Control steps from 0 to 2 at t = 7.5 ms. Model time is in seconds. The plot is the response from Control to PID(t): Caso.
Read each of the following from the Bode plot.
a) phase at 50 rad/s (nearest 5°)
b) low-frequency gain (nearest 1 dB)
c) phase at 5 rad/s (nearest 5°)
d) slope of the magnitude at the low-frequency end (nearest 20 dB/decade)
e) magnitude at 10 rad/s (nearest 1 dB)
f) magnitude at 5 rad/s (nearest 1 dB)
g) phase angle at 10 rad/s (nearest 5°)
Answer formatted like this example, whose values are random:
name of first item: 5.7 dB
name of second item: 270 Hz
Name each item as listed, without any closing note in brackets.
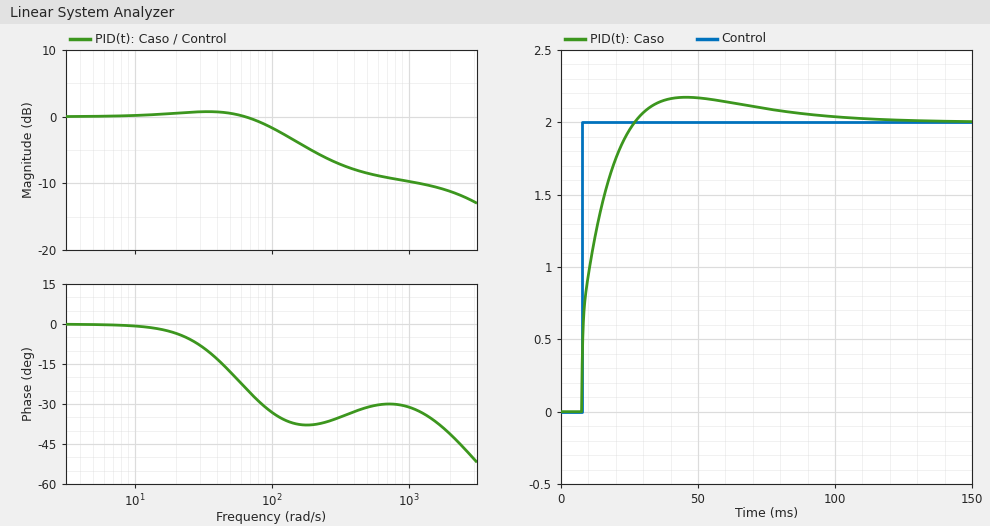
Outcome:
phase at 50 rad/s: -20°
low-frequency gain: 0 dB
phase at 5 rad/s: 0°
slope of the magnitude at the low-frequency end: 0 dB/decade
magnitude at 10 rad/s: 0 dB
magnitude at 5 rad/s: 0 dB
phase angle at 10 rad/s: 0°
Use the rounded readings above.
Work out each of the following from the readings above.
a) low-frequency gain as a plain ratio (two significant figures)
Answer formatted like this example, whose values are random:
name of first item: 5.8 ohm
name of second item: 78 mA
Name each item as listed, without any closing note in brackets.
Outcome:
low-frequency gain as a plain ratio: 1.0
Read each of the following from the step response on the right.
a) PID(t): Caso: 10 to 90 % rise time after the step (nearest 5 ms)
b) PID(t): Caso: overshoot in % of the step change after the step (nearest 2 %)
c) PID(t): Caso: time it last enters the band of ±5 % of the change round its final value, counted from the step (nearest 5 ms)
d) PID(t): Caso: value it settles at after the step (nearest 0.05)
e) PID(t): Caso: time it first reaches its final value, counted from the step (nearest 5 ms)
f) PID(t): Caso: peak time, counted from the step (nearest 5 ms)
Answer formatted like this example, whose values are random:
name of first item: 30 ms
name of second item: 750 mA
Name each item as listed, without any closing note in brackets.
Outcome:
PID(t): Caso: 10 to 90 % rise time after the step: 15 ms
PID(t): Caso: overshoot in % of the step change after the step: 8 %
PID(t): Caso: time it last enters the band of ±5 % of the change round its final value, counted from the step: 65 ms
PID(t): Caso: value it settles at after the step: 2.00
PID(t): Caso: time it first reaches its final value, counted from the step: 20 ms
PID(t): Caso: peak time, counted from the step: 40 ms
